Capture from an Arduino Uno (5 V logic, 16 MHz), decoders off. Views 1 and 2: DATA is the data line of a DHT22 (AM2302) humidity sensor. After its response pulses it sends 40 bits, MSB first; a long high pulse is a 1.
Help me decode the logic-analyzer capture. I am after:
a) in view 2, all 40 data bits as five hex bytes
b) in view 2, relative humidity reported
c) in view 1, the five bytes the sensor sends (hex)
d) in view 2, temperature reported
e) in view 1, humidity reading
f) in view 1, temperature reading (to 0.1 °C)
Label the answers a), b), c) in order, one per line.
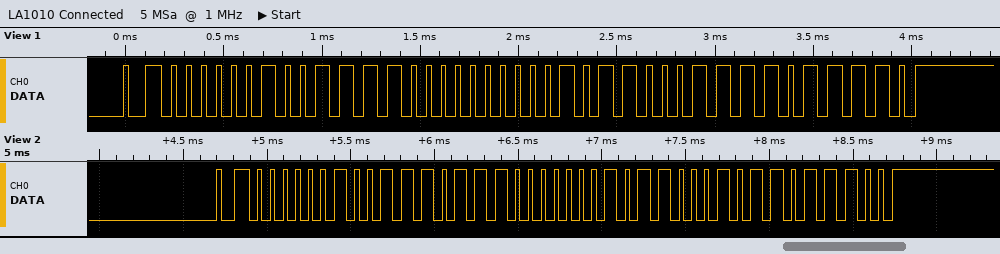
a) 02 77 01 62 DC
b) 63.1 %
c) 02 78 01 63 DE
d) 35.4 °C
e) 63.2 %
f) 35.5 °C
